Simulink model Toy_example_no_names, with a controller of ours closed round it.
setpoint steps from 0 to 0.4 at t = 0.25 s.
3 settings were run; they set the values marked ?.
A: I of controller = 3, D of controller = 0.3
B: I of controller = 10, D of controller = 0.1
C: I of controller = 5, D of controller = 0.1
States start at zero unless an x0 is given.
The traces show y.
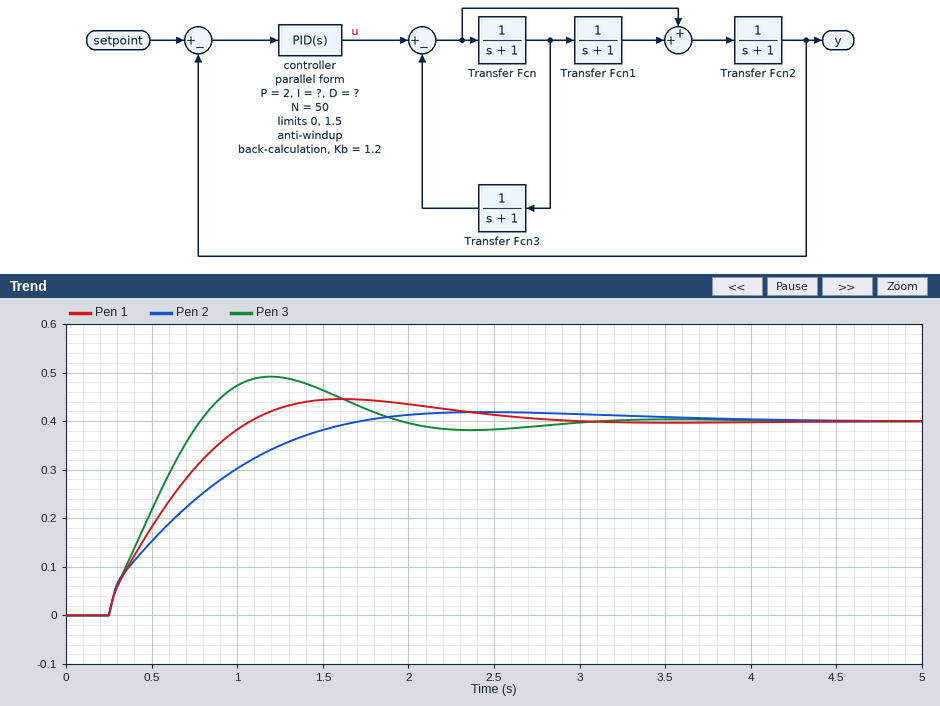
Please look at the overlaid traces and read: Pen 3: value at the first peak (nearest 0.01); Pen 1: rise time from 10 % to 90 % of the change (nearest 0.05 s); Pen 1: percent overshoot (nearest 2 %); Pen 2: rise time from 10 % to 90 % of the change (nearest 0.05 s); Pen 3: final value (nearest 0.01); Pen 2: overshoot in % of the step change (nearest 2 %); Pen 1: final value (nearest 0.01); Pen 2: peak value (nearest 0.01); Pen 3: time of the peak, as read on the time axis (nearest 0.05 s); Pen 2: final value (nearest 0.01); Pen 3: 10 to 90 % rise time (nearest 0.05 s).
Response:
0.49
0.65 s
12 %
1.05 s
0.40
4 %
0.40
0.42
1.20 s
0.40
0.45 s
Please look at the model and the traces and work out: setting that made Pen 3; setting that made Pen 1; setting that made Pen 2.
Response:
B
C
A
